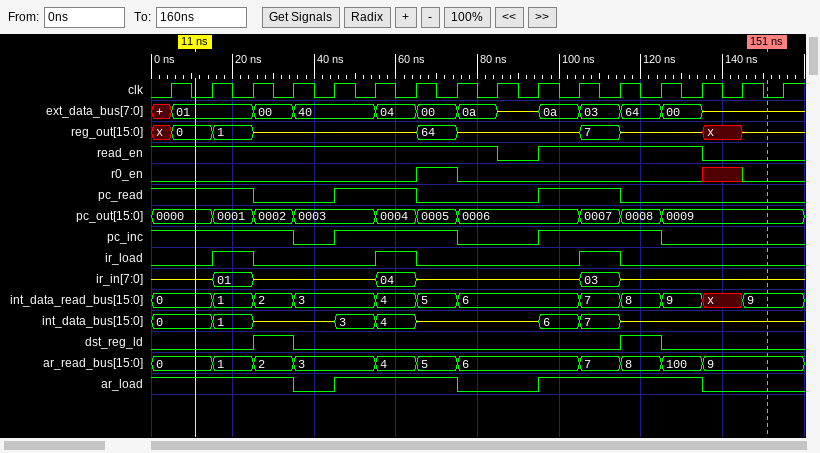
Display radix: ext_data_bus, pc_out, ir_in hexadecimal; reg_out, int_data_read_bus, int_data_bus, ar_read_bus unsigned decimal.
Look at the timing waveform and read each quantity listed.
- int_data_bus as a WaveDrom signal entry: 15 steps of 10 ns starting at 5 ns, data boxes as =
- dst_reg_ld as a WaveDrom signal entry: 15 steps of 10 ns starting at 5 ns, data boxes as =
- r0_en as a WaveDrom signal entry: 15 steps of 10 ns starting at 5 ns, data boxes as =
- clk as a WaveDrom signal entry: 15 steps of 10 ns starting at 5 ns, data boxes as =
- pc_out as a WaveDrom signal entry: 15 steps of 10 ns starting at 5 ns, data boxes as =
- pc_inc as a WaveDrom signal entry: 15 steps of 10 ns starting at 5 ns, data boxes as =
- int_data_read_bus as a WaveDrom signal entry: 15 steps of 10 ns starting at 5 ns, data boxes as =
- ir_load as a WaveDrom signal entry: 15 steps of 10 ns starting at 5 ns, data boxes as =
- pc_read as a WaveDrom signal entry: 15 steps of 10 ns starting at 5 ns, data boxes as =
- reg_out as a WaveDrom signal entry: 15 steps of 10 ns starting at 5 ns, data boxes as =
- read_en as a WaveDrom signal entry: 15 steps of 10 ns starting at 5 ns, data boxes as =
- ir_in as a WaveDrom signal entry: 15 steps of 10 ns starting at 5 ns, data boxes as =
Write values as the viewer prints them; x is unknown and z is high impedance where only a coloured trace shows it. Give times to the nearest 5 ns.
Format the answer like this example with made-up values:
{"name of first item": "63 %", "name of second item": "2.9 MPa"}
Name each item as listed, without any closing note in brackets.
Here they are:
{"int_data_bus as a WaveDrom signal entry: 15 steps of 10 ns starting at 5 ns, data boxes as =": "{name: 'int_data_bus', wave: '==z.==z..==z...', data: '0 1 3 4 6 7'}", "dst_reg_ld as a WaveDrom signal entry: 15 steps of 10 ns starting at 5 ns, data boxes as =": "{name: 'dst_reg_ld', wave: '0.10.......10..'}", "r0_en as a WaveDrom signal entry: 15 steps of 10 ns starting at 5 ns, data boxes as =": "{name: 'r0_en', wave: '0.....10.....x0'}", "clk as a WaveDrom signal entry: 15 steps of 10 ns starting at 5 ns, data boxes as =": "{name: 'clk', wave: 'p..............'}", "pc_out as a WaveDrom signal entry: 15 steps of 10 ns starting at 5 ns, data boxes as =": "{name: 'pc_out', wave: '====.===..===..', data: '0000 0001 0002 0003 0004 0005 0006 0007 0008 0009'}", "pc_inc as a WaveDrom signal entry: 15 steps of 10 ns starting at 5 ns, data boxes as =": "{name: 'pc_inc', wave: '1..01..0.1..0..'}", "int_data_read_bus as a WaveDrom signal entry: 15 steps of 10 ns starting at 5 ns, data boxes as =": "{name: 'int_data_read_bus', wave: '====.===..===x=', data: '0 1 2 3 4 5 6 7 8 9 9'}", "ir_load as a WaveDrom signal entry: 15 steps of 10 ns starting at 5 ns, data boxes as =": "{name: 'ir_load', wave: '010..10...10...'}", "pc_read as a WaveDrom signal entry: 15 steps of 10 ns starting at 5 ns, data boxes as =": "{name: 'pc_read', wave: '1.0.1.0..1.0...'}", "reg_out as a WaveDrom signal entry: 15 steps of 10 ns starting at 5 ns, data boxes as =": "{name: 'reg_out', wave: '==z...=z..=z.xz', data: '0 1 64 7'}", "read_en as a WaveDrom signal entry: 15 steps of 10 ns starting at 5 ns, data boxes as =": "{name: 'read_en', wave: '1.......01...0.'}", "ir_in as a WaveDrom signal entry: 15 steps of 10 ns starting at 5 ns, data boxes as =": "{name: 'ir_in', wave: 'z=z..=z...=z...', data: '01 04 03'}"}
